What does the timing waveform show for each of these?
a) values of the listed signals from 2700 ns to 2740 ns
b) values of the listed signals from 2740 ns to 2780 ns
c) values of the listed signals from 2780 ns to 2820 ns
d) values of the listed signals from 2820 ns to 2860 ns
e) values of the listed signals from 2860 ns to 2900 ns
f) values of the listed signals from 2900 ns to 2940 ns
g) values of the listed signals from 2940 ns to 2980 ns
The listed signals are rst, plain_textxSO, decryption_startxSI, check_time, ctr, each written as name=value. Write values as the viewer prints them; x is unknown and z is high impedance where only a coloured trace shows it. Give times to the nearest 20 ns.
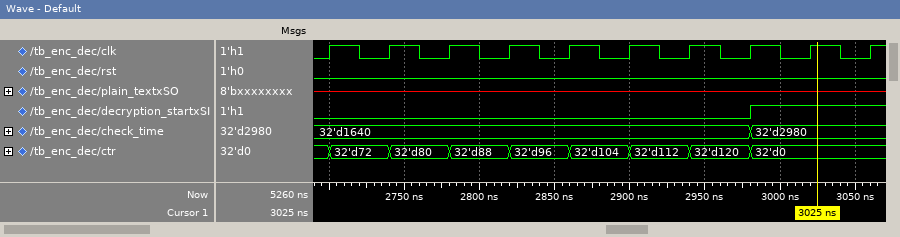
rst=0, plain_textxSO=x, decryption_startxSI=0, check_time=32'd1640, ctr=32'd72
rst=0, plain_textxSO=x, decryption_startxSI=0, check_time=32'd1640, ctr=32'd80
rst=0, plain_textxSO=x, decryption_startxSI=0, check_time=32'd1640, ctr=32'd88
rst=0, plain_textxSO=x, decryption_startxSI=0, check_time=32'd1640, ctr=32'd96
rst=0, plain_textxSO=x, decryption_startxSI=0, check_time=32'd1640, ctr=32'd104
rst=0, plain_textxSO=x, decryption_startxSI=0, check_time=32'd1640, ctr=32'd112
rst=0, plain_textxSO=x, decryption_startxSI=0, check_time=32'd1640, ctr=32'd120
